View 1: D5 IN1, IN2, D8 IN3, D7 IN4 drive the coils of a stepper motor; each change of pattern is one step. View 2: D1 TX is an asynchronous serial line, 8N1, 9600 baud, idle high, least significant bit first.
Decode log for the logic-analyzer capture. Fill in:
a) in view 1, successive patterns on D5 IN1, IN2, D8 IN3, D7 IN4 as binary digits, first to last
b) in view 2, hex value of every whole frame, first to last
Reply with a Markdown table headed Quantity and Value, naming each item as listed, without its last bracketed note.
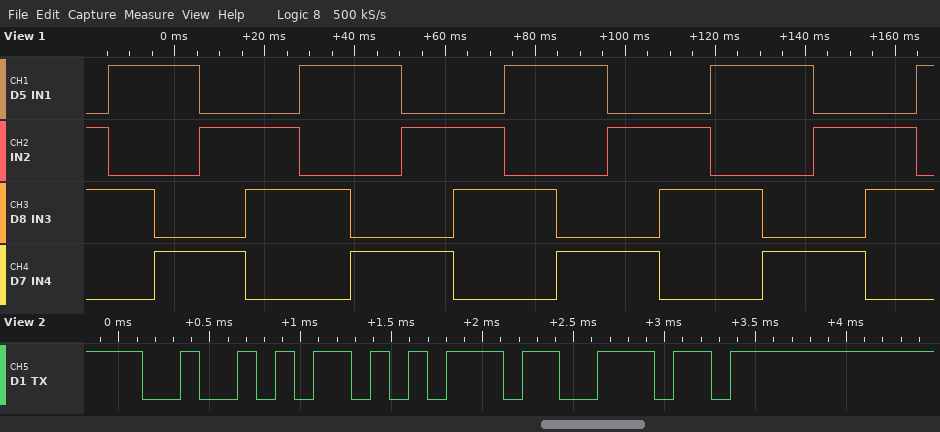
| Quantity | Value |
|---|---|
| in view 1, successive patterns on D5 IN1, IN2, D8 IN3, D7 IN4 as binary digits, first to last | 0110 1010 1001 0101 0110 1010 1001 0101 0110 1010 1001 0101 0110 1010 1001 0101 0110 1010 |
| in view 2, hex value of every whole frame, first to last | 52 75 6E |
